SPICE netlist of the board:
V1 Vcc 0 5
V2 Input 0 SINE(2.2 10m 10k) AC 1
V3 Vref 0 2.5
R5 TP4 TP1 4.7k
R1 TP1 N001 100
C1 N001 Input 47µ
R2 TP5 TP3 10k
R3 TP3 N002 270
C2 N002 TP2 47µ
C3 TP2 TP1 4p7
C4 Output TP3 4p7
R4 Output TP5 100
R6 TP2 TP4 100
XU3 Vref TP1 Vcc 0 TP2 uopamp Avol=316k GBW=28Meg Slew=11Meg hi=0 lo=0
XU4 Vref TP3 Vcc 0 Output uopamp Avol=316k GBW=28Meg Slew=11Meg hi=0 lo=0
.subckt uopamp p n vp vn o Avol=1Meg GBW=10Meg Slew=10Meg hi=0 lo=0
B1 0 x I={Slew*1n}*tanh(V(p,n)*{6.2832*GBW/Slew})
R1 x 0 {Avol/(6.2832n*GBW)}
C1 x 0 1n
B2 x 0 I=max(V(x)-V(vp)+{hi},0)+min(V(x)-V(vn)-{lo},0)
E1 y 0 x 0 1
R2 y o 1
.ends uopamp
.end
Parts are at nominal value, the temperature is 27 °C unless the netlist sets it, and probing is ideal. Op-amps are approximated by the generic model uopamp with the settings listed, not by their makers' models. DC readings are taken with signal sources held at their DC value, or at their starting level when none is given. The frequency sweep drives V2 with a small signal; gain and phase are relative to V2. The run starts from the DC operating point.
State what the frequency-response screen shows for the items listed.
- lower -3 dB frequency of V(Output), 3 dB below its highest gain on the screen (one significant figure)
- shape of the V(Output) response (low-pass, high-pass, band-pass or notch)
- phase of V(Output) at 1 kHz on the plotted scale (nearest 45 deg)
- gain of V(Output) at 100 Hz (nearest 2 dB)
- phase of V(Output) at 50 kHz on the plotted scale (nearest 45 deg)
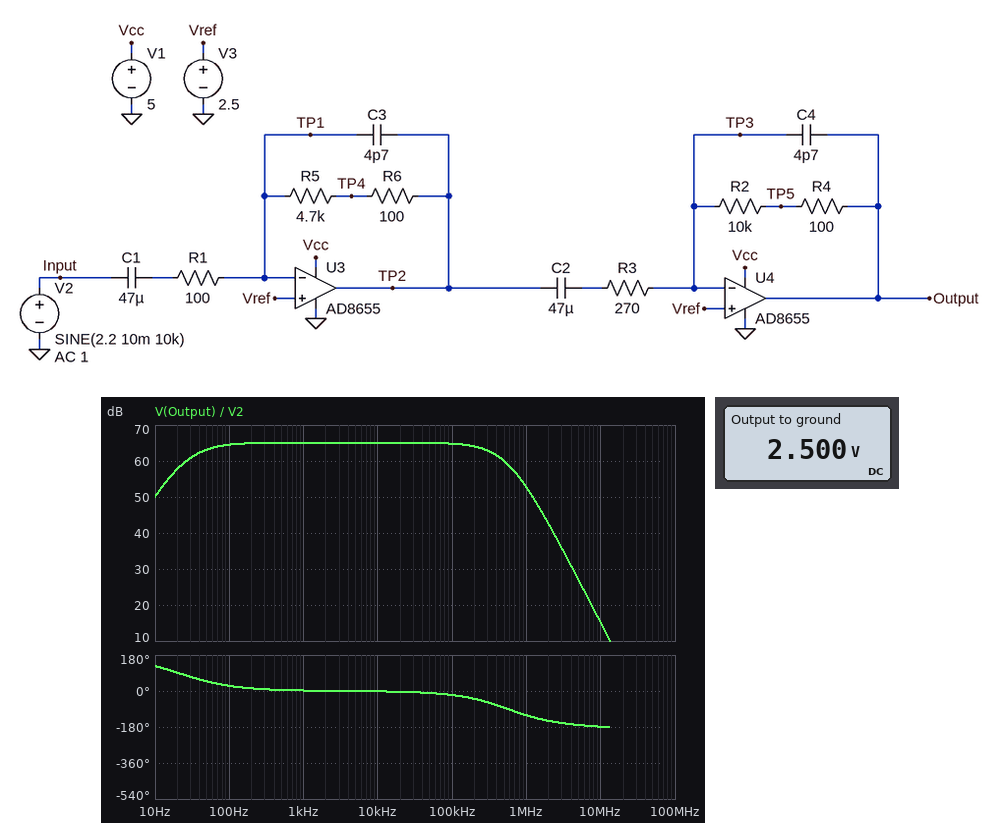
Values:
40 Hz
band-pass
0 deg
64 dB
0 deg
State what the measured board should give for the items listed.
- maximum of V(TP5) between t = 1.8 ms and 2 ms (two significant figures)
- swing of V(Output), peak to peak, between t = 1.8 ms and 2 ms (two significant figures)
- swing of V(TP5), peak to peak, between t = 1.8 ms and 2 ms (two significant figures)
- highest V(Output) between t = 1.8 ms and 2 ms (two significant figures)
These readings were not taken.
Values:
5.0 V
5.0 V
5.0 V
5.0 V
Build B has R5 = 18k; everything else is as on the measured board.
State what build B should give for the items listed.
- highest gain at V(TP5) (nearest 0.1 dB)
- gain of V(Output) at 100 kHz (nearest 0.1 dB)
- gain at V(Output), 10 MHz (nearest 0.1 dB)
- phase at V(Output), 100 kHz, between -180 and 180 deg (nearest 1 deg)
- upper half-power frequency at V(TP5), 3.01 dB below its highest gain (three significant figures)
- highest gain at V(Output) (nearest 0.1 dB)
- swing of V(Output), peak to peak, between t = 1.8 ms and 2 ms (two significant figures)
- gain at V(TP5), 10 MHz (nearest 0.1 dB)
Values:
76.5 dB
74.7 dB
15.2 dB
-45 deg
135 kHz
76.6 dB
5.0 V
15.1 dB
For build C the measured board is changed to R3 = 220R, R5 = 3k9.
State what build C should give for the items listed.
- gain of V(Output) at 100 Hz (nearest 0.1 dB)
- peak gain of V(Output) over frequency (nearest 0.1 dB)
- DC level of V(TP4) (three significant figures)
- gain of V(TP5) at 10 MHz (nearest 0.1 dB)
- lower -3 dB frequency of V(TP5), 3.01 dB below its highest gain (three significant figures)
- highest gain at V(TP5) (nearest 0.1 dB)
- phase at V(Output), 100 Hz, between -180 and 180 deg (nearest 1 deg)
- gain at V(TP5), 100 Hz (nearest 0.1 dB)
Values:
64.7 dB
65.3 dB
2.50 V
15.3 dB
39.5 Hz
65.2 dB
27 deg
64.6 dB
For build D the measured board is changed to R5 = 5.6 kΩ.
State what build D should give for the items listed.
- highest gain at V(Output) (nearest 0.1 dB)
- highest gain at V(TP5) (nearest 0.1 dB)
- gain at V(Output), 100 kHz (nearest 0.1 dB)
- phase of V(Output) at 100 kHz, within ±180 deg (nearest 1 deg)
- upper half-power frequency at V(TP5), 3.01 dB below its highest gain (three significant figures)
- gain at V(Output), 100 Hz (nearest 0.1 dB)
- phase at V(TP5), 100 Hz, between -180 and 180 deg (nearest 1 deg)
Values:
66.6 dB
66.5 dB
66.2 dB
-22 deg
328 kHz
66.0 dB
26 deg
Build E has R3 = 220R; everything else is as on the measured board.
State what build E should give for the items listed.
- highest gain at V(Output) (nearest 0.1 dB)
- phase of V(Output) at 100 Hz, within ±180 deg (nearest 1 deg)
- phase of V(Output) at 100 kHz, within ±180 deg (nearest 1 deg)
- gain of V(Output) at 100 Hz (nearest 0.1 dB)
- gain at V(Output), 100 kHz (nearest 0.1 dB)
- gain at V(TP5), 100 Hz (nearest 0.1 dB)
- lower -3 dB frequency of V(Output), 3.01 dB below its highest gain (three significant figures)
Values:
66.9 dB
27 deg
-22 deg
66.3 dB
66.5 dB
66.2 dB
39.5 Hz
